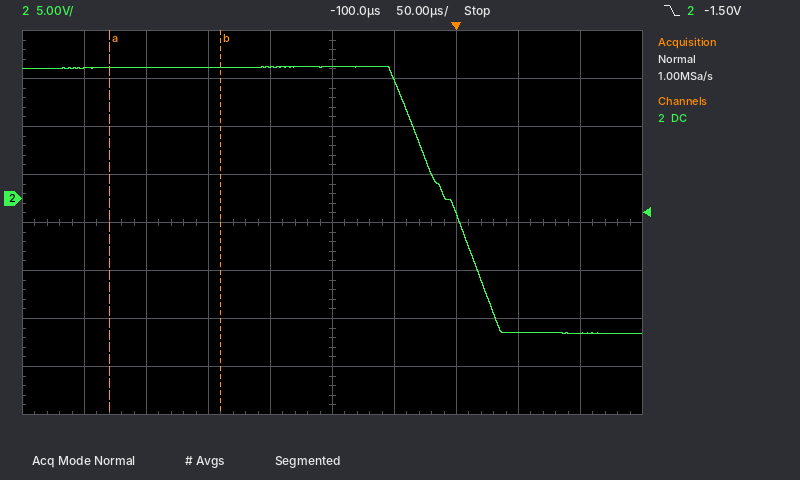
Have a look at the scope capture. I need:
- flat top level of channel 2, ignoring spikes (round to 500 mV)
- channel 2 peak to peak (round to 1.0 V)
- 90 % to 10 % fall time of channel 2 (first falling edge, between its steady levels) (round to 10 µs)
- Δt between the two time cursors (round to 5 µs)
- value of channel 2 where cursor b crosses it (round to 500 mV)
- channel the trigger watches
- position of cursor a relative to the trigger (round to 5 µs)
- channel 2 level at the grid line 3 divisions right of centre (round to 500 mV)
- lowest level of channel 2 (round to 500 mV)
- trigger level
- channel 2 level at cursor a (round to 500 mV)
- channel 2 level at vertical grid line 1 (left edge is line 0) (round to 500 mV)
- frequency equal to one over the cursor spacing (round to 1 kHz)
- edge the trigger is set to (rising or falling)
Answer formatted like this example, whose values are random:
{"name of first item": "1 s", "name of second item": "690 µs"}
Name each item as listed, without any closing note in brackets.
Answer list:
{"flat top level of channel 2, ignoring spikes": "13.5 V", "channel 2 peak to peak": "28.0 V", "90 % to 10 % fall time of channel 2 (first falling edge, between its steady levels)": "70 µs", "Δt between the two time cursors": "90 µs", "value of channel 2 where cursor b crosses it": "13.5 V", "channel the trigger watches": "channel 2", "position of cursor a relative to the trigger": "-280 µs", "channel 2 level at the grid line 3 divisions right of centre": "-14.0 V", "lowest level of channel 2": "-14.0 V", "trigger level": "-1.50 V", "channel 2 level at cursor a": "13.5 V", "channel 2 level at vertical grid line 1 (left edge is line 0)": "13.5 V", "frequency equal to one over the cursor spacing": "11 kHz", "edge the trigger is set to": "falling"}
